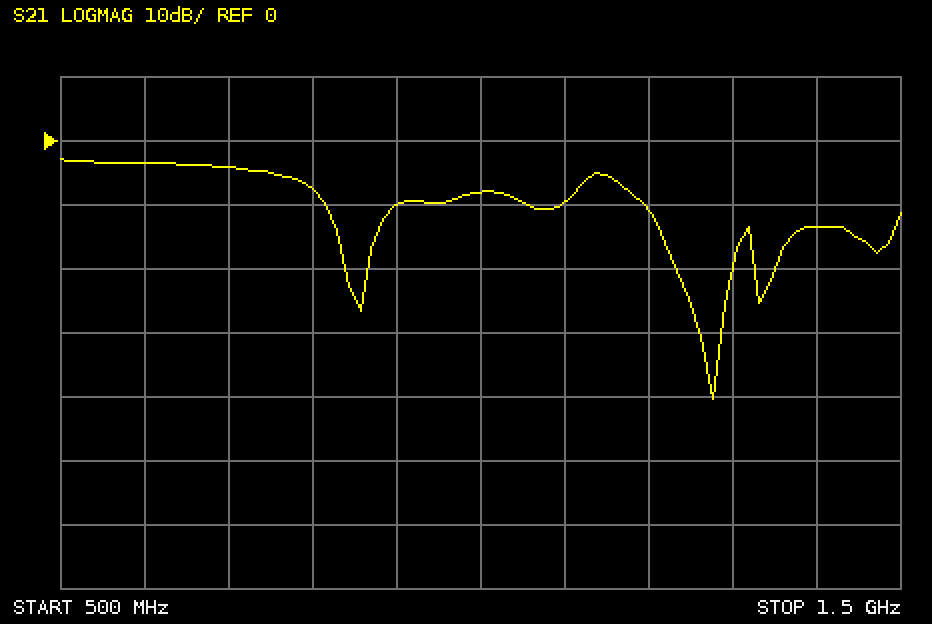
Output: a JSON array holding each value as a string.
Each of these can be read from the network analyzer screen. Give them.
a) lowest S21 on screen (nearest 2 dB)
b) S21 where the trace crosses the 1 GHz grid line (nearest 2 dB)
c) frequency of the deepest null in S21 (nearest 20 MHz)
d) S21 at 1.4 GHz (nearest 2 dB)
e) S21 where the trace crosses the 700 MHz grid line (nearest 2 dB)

["-40 dB", "-8 dB", "1.28 GHz", "-14 dB", "-4 dB"]
